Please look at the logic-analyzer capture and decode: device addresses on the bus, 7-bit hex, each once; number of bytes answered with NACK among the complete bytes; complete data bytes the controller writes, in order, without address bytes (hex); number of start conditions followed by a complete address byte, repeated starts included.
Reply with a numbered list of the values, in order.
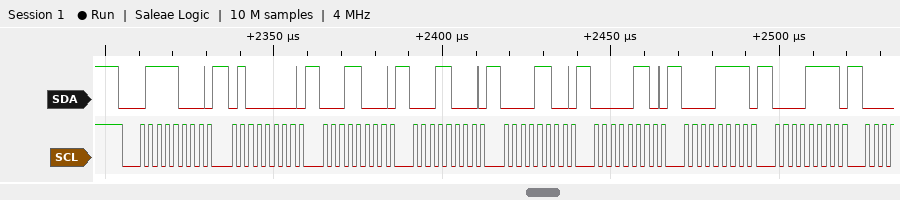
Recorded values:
1. 0x3C
2. 0
3. 40 18 18 0C 06 0F 0F
4. 1
